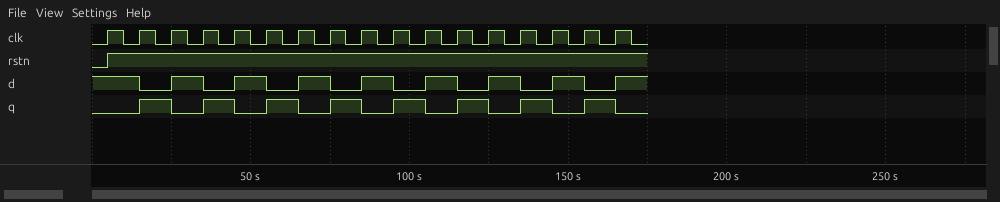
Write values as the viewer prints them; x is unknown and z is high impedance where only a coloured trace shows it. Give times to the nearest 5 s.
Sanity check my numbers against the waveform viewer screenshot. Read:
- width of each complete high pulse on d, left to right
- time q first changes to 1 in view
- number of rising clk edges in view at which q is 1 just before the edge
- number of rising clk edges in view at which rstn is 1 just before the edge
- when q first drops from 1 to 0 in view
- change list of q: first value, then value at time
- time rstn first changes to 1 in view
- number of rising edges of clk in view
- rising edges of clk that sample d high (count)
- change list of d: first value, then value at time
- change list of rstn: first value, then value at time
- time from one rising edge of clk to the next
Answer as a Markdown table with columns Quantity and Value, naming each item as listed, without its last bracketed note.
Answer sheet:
| Quantity | Value |
|---|---|
| width of each complete high pulse on d, left to right | 10 s, 10 s, 10 s, 10 s, 10 s, 10 s, 10 s |
| time q first changes to 1 in view | 15 s |
| number of rising clk edges in view at which q is 1 just before the edge | 8 |
| number of rising clk edges in view at which rstn is 1 just before the edge | 16 |
| when q first drops from 1 to 0 in view | 25 s |
| change list of q: first value, then value at time | 0, 1 at 15 s, 0 at 25 s, 1 at 35 s, 0 at 45 s, 1 at 55 s, 0 at 65 s, 1 at 75 s, 0 at 85 s, 1 at 95 s, 0 at 105 s, 1 at 115 s, 0 at 125 s, 1 at 135 s, 0 at 145 s, 1 at 155 s, 0 at 165 s |
| time rstn first changes to 1 in view | 5 s |
| number of rising edges of clk in view | 17 |
| rising edges of clk that sample d high | 9 |
| change list of d: first value, then value at time | 1, 0 at 15 s, 1 at 25 s, 0 at 35 s, 1 at 45 s, 0 at 55 s, 1 at 65 s, 0 at 75 s, 1 at 85 s, 0 at 95 s, 1 at 105 s, 0 at 115 s, 1 at 125 s, 0 at 135 s, 1 at 145 s, 0 at 155 s, 1 at 165 s |
| change list of rstn: first value, then value at time | 0, 1 at 5 s |
| time from one rising edge of clk to the next | 10 s |
